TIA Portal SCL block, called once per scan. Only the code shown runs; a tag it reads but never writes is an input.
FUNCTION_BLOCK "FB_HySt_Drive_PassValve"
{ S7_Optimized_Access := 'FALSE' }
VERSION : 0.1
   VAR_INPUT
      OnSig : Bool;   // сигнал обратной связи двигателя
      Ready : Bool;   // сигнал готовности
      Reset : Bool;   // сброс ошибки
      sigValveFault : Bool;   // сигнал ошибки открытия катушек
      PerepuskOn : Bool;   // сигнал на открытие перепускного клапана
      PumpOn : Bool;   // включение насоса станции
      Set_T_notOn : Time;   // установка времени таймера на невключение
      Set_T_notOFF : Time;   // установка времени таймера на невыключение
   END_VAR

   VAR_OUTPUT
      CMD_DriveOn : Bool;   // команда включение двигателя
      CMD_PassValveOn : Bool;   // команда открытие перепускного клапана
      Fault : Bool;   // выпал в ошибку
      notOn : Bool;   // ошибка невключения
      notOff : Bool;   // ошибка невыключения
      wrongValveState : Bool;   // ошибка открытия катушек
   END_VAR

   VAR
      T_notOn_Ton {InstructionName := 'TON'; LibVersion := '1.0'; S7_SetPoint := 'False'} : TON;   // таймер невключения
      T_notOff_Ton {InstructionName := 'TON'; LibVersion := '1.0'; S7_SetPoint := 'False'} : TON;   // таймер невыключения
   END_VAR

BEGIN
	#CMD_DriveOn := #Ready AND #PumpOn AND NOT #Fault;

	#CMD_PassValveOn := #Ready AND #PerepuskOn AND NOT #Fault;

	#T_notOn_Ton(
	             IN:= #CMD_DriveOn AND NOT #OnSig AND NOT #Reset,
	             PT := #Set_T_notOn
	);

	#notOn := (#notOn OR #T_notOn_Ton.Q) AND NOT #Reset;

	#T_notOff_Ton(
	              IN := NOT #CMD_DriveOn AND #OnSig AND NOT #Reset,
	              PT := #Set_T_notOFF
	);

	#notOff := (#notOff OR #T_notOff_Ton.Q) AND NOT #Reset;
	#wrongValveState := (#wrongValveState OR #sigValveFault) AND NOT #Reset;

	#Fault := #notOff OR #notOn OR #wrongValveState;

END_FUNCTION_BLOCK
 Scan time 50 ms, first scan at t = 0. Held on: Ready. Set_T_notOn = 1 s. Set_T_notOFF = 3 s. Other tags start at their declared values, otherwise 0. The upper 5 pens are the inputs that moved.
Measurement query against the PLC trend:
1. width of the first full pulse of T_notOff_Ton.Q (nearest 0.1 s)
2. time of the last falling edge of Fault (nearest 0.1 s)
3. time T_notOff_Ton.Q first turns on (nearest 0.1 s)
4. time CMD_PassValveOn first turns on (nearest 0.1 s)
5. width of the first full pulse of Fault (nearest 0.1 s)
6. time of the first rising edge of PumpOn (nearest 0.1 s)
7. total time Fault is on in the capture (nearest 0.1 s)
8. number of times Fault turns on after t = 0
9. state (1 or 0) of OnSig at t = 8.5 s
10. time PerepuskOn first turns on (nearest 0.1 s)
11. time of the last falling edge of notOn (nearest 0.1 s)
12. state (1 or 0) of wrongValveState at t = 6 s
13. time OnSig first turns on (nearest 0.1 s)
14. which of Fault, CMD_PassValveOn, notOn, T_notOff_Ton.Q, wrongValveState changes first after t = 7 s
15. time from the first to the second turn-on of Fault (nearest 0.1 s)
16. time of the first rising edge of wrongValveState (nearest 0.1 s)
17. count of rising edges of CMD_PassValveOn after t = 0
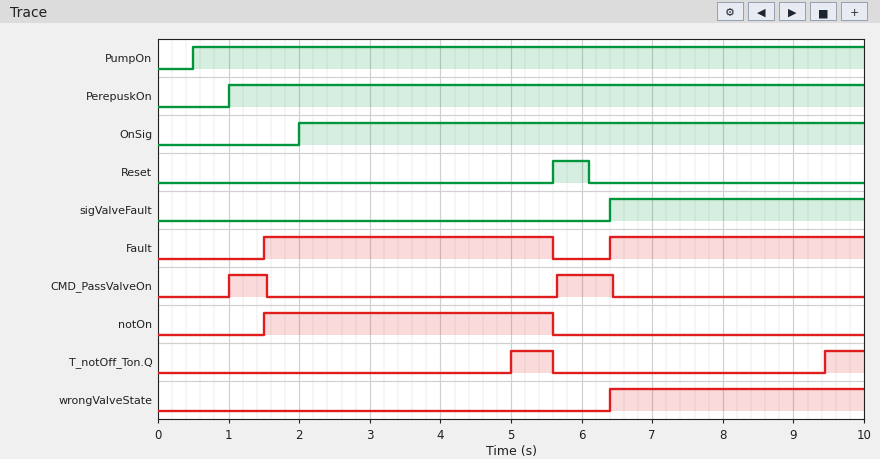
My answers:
0.6 s
5.6 s
5.0 s
1.0 s
4.1 s
0.5 s
7.7 s
2
1
1.0 s
5.6 s
0
2.0 s
T_notOff_Ton.Q
4.9 s
6.4 s
2
